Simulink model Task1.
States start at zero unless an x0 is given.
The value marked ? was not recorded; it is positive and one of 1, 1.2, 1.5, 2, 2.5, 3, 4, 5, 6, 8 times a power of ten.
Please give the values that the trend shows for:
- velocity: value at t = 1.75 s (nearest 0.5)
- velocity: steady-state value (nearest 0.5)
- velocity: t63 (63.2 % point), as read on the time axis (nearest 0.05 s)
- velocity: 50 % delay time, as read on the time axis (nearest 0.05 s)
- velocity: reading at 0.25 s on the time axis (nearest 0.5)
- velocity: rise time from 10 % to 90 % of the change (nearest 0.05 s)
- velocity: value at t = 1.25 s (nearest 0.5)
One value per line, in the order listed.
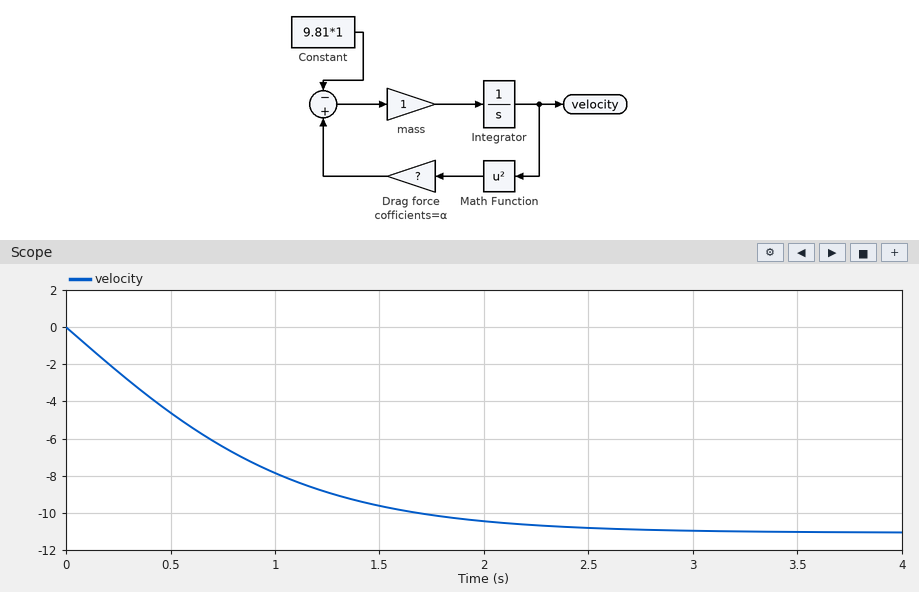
-10.0
-11.0
0.85 s
0.60 s
-2.5
1.55 s
-9.0
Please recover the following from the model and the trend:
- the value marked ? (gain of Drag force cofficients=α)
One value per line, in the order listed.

0.08
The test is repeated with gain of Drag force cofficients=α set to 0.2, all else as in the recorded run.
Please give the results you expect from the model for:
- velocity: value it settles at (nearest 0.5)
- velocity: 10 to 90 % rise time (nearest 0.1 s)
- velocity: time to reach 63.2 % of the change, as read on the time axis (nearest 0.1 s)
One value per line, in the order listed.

-7.0
1.0 s
0.5 s
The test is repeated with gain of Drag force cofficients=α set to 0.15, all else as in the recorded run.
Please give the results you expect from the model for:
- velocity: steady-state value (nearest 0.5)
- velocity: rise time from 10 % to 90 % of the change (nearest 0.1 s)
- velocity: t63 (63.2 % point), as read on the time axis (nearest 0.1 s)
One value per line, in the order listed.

-8.0
1.1 s
0.6 s
